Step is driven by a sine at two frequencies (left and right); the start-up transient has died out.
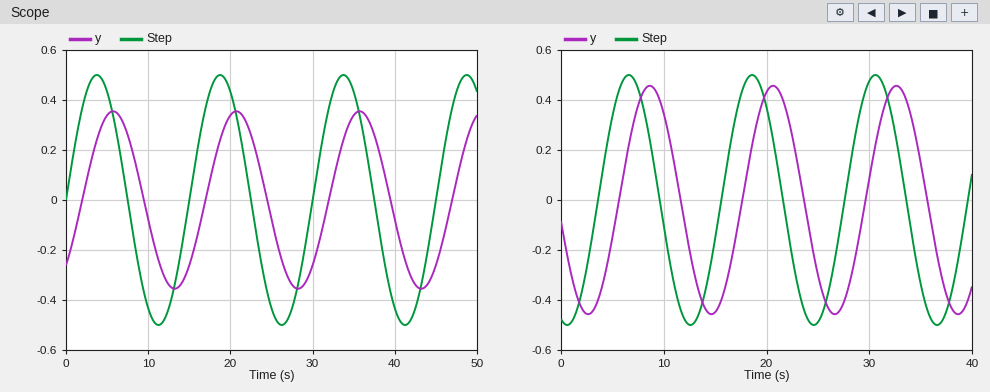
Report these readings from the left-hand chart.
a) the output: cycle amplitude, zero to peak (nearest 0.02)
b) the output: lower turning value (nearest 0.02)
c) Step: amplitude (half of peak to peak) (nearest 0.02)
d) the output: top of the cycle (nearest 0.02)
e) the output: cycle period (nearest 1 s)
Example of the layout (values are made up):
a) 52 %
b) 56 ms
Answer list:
a) 0.36
b) -0.36
c) 0.50
d) 0.36
e) 15 s
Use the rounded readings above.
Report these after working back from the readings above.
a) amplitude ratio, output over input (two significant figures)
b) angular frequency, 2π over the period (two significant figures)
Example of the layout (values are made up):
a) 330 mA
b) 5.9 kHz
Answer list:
a) 0.72
b) 0.42 rad/s
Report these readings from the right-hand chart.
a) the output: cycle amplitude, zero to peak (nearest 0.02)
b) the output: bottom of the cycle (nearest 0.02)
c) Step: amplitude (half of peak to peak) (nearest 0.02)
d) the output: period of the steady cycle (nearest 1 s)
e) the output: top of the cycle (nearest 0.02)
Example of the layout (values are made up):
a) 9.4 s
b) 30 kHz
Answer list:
a) 0.46
b) -0.46
c) 0.50
d) 12 s
e) 0.46
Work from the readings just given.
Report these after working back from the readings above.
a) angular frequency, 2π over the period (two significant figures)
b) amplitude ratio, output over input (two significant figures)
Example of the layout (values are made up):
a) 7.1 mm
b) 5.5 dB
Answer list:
a) 0.52 rad/s
b) 0.92
